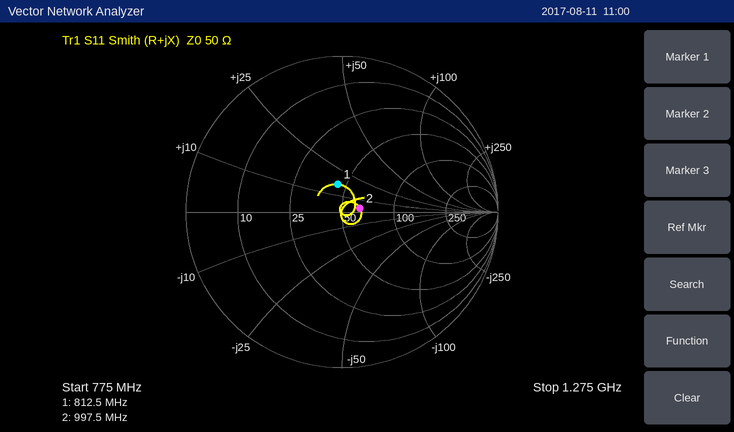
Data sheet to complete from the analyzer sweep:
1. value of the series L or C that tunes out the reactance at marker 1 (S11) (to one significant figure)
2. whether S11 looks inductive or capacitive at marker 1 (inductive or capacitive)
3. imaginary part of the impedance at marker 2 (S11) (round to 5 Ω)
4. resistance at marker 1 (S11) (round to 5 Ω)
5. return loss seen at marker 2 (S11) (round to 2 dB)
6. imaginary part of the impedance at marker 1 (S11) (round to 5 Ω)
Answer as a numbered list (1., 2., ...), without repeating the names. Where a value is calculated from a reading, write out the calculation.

1. C = 1/(2π × 812.5 MHz × 15 Ω) ≈ 13.1 pF, so 10 pF to one significant figure
2. inductive
3. +5 Ω
4. 45 Ω
5. 18 dB
6. +15 Ω
